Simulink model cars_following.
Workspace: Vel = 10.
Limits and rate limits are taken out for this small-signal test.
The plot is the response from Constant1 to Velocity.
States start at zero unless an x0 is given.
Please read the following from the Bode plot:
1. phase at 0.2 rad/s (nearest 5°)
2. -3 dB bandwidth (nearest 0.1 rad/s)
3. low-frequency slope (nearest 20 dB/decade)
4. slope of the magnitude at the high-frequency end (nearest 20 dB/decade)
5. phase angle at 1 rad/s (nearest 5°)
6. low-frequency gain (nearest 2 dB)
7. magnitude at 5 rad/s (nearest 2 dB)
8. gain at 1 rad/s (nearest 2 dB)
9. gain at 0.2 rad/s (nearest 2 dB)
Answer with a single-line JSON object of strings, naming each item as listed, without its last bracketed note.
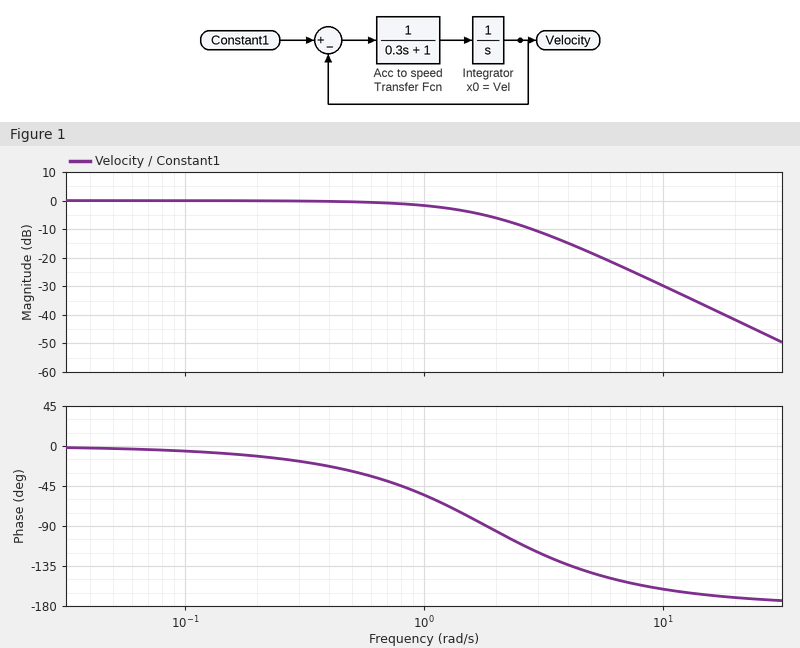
{"phase at 0.2 rad/s": "-10°", "-3 dB bandwidth": "1.3 rad/s", "low-frequency slope": "0 dB/decade", "slope of the magnitude at the high-frequency end": "-40 dB/decade", "phase angle at 1 rad/s": "-55°", "low-frequency gain": "0 dB", "magnitude at 5 rad/s": "-18 dB", "gain at 1 rad/s": "-2 dB", "gain at 0.2 rad/s": "0 dB"}
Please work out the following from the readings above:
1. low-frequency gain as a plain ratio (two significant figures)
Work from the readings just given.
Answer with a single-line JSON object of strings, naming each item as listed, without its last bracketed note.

{"low-frequency gain as a plain ratio": "1.0"}
